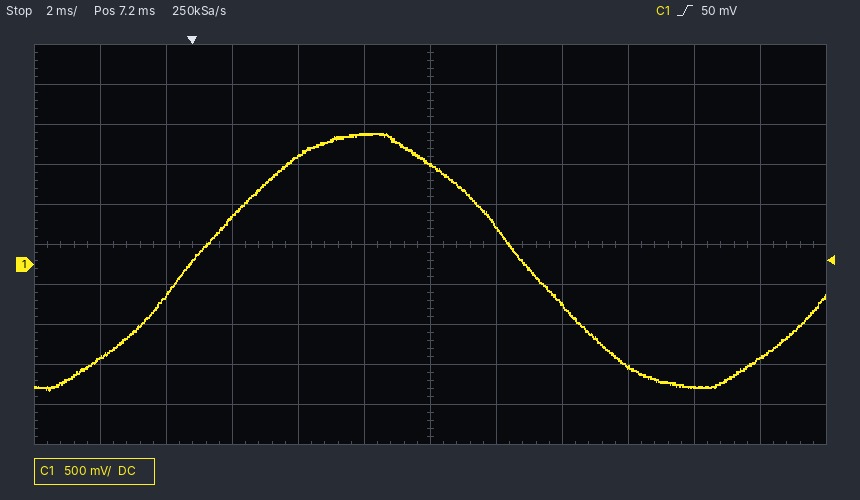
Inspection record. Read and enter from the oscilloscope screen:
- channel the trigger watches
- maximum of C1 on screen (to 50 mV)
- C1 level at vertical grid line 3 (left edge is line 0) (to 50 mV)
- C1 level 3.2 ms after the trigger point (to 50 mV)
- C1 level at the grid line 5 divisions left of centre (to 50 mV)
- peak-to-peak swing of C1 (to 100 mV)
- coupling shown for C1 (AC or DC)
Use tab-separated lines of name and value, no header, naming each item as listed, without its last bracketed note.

channel the trigger watches	C1
maximum of C1 on screen	1.65 V
C1 level at vertical grid line 3 (left edge is line 0)	600 mV
C1 level 3.2 ms after the trigger point	1.35 V
C1 level at the grid line 5 divisions left of centre	-1.15 V
peak-to-peak swing of C1	3.20 V
coupling shown for C1	DC
